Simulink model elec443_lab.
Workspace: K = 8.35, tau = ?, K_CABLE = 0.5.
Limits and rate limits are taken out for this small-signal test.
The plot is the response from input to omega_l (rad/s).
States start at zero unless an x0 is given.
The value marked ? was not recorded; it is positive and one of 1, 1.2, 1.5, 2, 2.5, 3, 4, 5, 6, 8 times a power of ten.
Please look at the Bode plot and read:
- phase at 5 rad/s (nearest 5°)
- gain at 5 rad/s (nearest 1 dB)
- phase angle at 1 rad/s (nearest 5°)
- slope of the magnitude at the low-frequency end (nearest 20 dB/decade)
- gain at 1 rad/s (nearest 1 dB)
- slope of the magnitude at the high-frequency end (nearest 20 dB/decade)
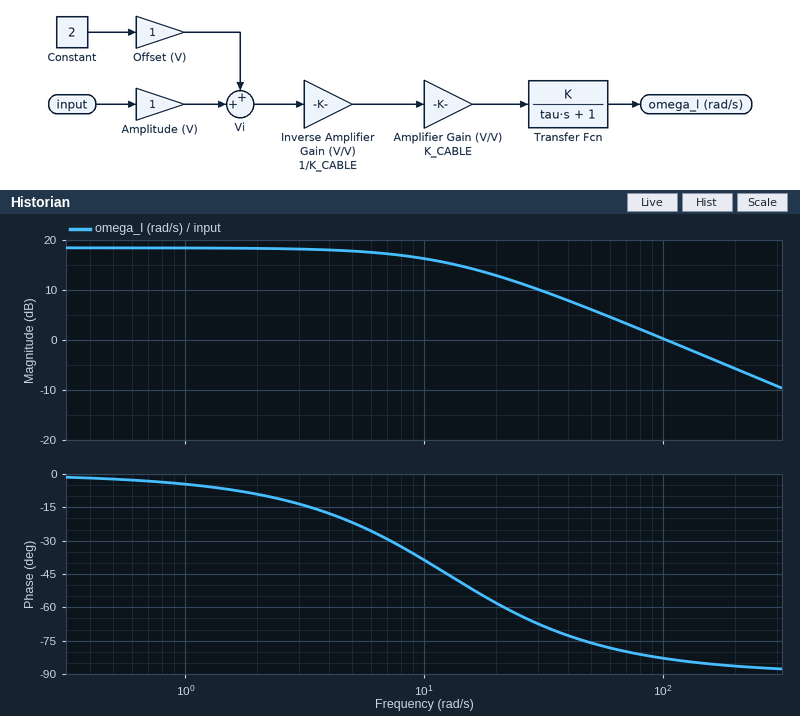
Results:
-20°
18 dB
-5°
0 dB/decade
18 dB
-20 dB/decade
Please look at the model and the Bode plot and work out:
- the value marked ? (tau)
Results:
0.08
